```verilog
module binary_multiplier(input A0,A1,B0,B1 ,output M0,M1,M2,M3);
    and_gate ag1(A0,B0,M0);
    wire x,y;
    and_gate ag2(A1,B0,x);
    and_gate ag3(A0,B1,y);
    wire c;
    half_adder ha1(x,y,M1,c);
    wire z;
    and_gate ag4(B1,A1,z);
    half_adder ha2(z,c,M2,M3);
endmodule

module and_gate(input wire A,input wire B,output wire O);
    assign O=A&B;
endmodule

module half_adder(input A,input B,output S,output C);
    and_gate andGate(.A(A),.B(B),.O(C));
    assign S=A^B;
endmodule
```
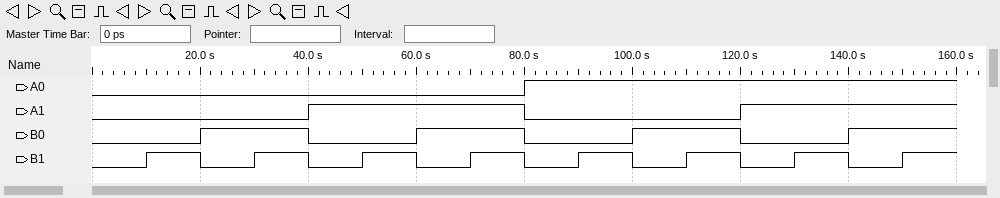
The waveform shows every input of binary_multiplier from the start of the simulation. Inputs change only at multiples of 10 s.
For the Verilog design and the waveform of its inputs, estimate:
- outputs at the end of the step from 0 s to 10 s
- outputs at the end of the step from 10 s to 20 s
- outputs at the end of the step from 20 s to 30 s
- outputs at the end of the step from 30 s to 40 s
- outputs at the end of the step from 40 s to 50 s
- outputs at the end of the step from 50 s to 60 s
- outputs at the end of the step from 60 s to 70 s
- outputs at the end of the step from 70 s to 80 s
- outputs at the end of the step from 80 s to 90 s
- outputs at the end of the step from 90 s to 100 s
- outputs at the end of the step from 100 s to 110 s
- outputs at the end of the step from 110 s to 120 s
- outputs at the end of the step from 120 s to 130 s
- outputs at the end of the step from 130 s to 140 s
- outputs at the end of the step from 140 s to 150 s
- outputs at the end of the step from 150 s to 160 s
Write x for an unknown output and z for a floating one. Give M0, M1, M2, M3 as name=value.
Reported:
M0=0, M1=0, M2=0, M3=0
M0=0, M1=0, M2=0, M3=0
M0=0, M1=0, M2=0, M3=0
M0=0, M1=0, M2=0, M3=0
M0=0, M1=0, M2=0, M3=0
M0=0, M1=0, M2=1, M3=0
M0=0, M1=1, M2=0, M3=0
M0=0, M1=1, M2=1, M3=0
M0=0, M1=0, M2=0, M3=0
M0=0, M1=1, M2=0, M3=0
M0=1, M1=0, M2=0, M3=0
M0=1, M1=1, M2=0, M3=0
M0=0, M1=0, M2=0, M3=0
M0=0, M1=1, M2=1, M3=0
M0=1, M1=1, M2=0, M3=0
M0=1, M1=0, M2=0, M3=1
